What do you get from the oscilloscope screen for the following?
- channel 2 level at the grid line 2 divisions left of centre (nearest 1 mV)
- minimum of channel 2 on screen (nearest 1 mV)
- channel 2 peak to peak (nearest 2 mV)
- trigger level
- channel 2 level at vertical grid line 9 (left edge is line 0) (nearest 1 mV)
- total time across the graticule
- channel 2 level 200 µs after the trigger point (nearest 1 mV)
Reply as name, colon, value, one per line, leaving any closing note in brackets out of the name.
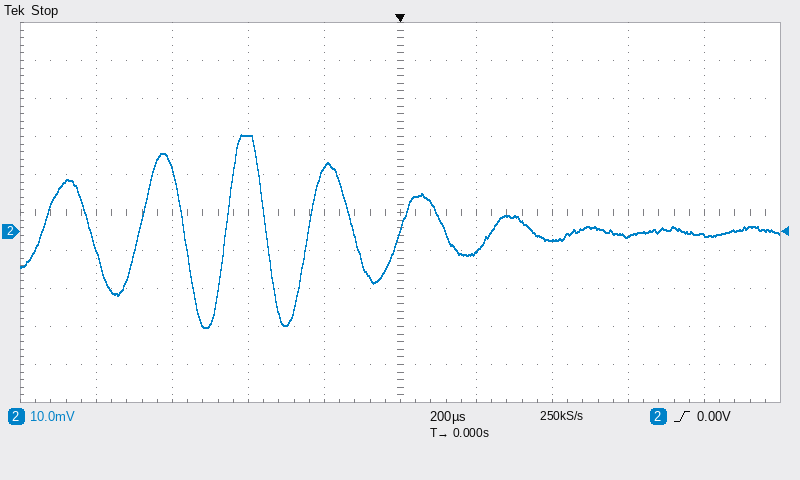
channel 2 level at the grid line 2 divisions left of centre: 25 mV
minimum of channel 2 on screen: -25 mV
channel 2 peak to peak: 50 mV
trigger level: 0.00 V
channel 2 level at vertical grid line 9 (left edge is line 0): -1 mV
total time across the graticule: 2 ms
channel 2 level 200 µs after the trigger point: -5 mV
